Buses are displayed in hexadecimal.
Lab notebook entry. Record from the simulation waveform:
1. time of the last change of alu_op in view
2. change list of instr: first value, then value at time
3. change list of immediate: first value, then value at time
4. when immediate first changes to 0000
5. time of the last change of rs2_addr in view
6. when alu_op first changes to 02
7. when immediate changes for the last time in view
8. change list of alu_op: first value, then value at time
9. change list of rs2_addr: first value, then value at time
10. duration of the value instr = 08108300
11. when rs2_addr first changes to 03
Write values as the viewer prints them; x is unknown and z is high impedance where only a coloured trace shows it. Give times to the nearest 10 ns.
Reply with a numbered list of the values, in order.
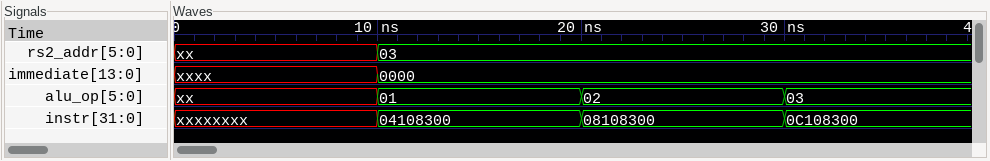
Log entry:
1. 30 ns
2. xxxxxxxx, 04108300 at 10 ns, 08108300 at 20 ns, 0C108300 at 30 ns
3. xxxx, 0000 at 10 ns
4. 10 ns
5. 10 ns
6. 20 ns
7. 10 ns
8. xx, 01 at 10 ns, 02 at 20 ns, 03 at 30 ns
9. xx, 03 at 10 ns
10. 10 ns
11. 10 ns
